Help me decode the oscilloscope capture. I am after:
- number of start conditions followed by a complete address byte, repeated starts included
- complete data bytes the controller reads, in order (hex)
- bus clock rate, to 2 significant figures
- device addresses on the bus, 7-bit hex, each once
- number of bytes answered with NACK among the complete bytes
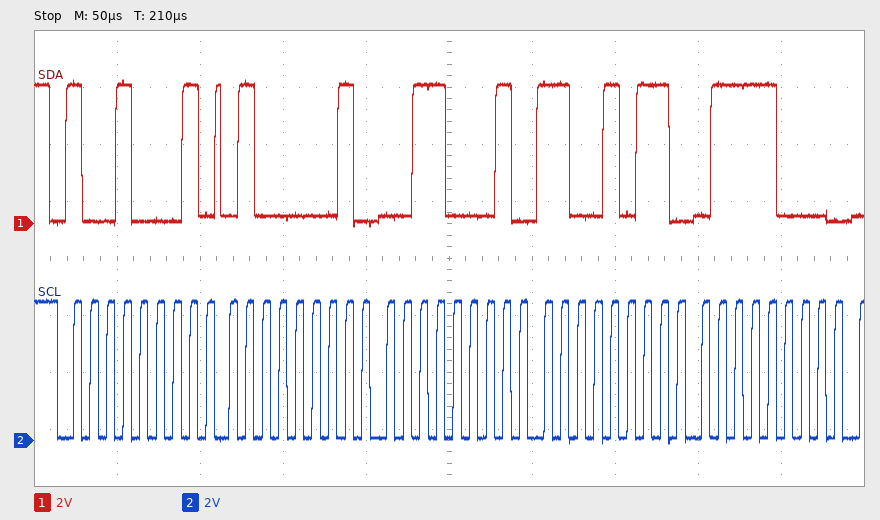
1
41 31 CB 78
100 kHz
0x48
0
